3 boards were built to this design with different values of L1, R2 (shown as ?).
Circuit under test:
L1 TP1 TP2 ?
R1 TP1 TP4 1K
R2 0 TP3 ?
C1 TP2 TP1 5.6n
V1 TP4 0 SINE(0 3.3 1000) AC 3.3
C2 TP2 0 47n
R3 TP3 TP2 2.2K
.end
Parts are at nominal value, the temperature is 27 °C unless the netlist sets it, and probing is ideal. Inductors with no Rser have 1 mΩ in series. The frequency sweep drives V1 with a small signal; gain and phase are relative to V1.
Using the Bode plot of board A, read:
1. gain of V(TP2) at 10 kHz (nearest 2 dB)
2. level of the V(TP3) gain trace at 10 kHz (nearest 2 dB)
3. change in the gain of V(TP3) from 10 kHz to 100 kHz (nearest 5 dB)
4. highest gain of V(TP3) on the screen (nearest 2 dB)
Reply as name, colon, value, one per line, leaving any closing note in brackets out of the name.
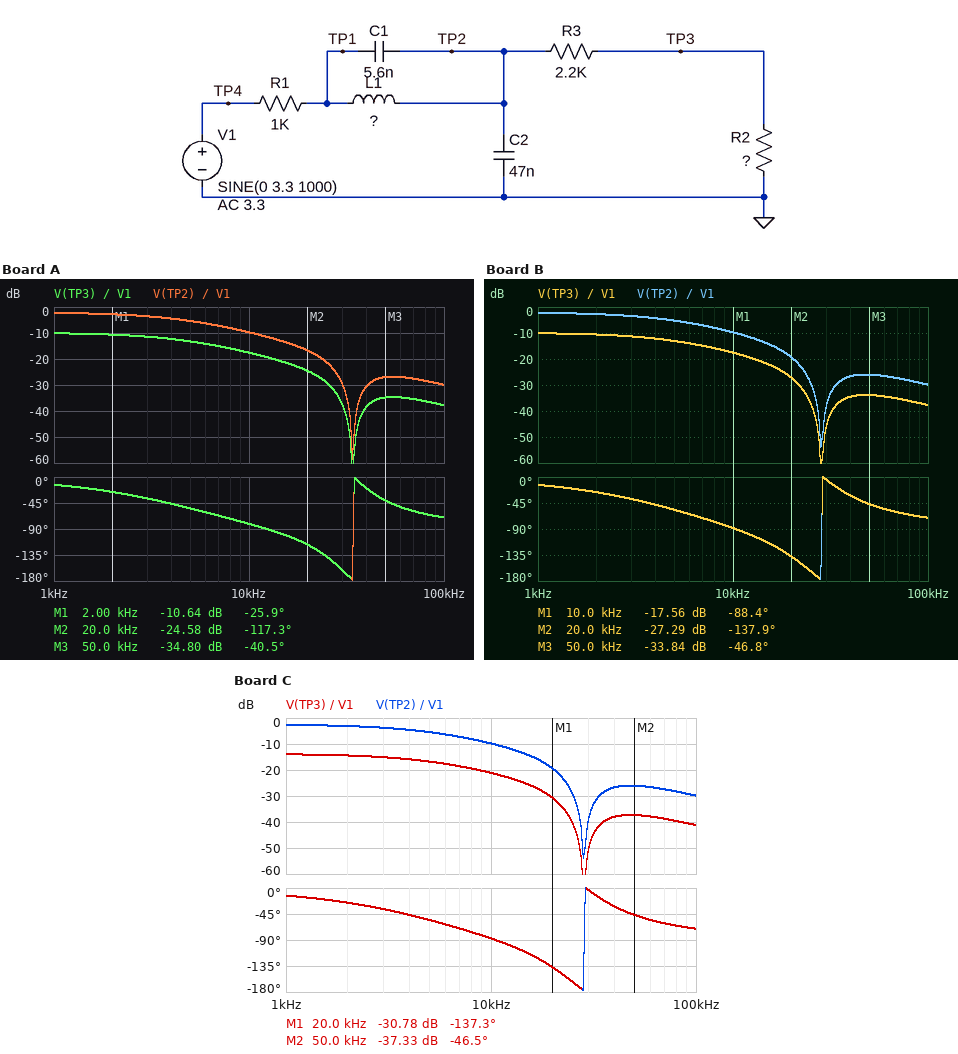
gain of V(TP2) at 10 kHz: -10 dB
level of the V(TP3) gain trace at 10 kHz: -18 dB
change in the gain of V(TP3) from 10 kHz to 100 kHz: -20 dB
highest gain of V(TP3) on the screen: -10 dB
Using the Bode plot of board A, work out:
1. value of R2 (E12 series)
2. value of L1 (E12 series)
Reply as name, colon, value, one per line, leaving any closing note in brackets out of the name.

value of R2: 1.5 kΩ
value of L1: 3.9 mH
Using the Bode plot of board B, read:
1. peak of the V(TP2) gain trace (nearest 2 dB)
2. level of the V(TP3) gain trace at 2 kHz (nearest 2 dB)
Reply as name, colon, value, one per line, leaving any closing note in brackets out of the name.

peak of the V(TP2) gain trace: -2 dB
level of the V(TP3) gain trace at 2 kHz: -10 dB
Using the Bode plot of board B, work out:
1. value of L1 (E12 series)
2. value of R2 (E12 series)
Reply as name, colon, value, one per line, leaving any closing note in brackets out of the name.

value of L1: 5.6 mH
value of R2: 1.5 kΩ
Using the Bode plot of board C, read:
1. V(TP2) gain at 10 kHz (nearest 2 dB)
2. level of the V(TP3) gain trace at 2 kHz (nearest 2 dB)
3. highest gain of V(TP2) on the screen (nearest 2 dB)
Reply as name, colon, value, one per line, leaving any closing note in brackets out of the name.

V(TP2) gain at 10 kHz: -10 dB
level of the V(TP3) gain trace at 2 kHz: -14 dB
highest gain of V(TP2) on the screen: -2 dB
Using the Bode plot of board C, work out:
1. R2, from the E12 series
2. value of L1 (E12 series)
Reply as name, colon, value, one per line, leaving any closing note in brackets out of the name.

R2, from the E12 series: 820 Ω
value of L1: 5.6 mH
